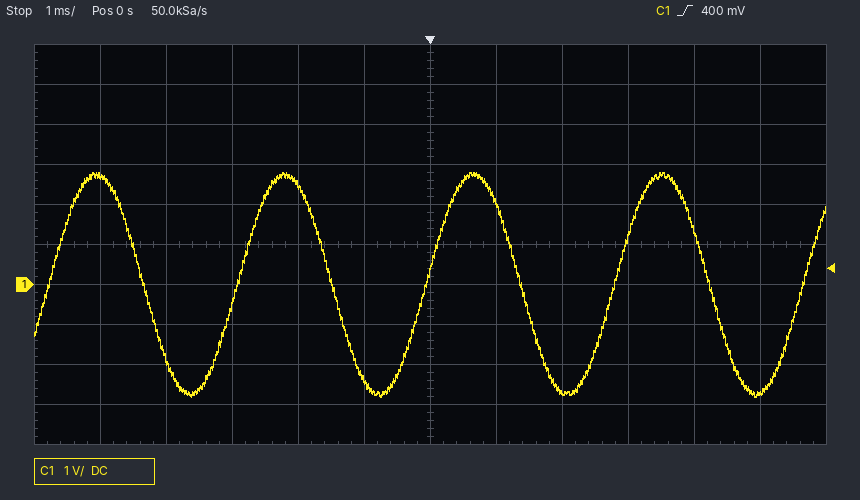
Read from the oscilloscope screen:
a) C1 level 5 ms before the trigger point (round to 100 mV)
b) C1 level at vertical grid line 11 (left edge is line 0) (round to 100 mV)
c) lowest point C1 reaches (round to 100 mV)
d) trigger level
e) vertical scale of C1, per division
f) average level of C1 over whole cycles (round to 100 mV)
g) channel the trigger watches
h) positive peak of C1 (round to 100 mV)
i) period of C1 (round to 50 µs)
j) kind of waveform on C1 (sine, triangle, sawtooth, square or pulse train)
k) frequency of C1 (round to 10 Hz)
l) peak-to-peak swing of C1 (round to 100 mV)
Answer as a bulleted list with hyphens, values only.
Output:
- 2.7 V
- -2.7 V
- -2.8 V
- 400 mV
- 1 V
- 0.0 V
- C1
- 2.8 V
- 2.85 ms
- sine
- 350 Hz
- 5.6 V
